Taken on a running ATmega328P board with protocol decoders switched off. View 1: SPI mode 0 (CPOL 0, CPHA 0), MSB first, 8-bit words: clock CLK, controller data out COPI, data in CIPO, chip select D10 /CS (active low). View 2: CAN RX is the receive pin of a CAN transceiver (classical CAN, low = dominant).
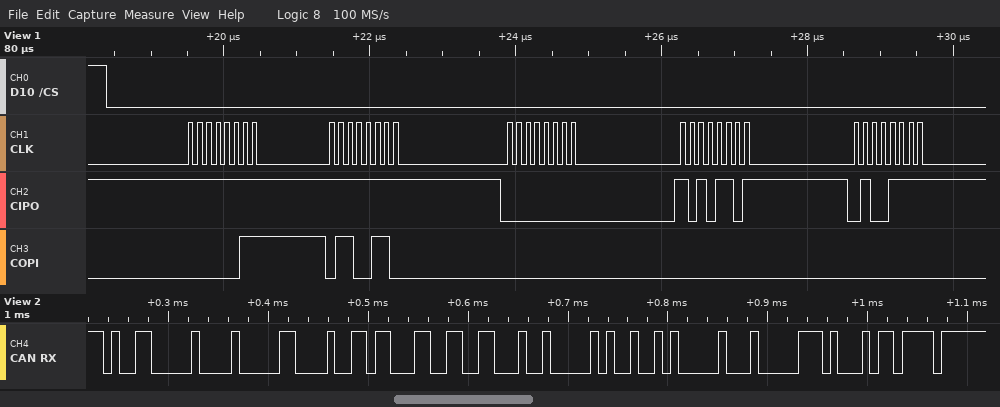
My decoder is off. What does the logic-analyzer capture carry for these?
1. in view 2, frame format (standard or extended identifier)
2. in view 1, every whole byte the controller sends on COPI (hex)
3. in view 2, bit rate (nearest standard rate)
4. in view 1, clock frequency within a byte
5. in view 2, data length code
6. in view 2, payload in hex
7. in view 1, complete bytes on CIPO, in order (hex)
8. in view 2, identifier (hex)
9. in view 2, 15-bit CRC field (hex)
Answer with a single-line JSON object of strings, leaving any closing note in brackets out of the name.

{"in view 2, frame format": "standard", "in view 1, every whole byte the controller sends on COPI": "0x03 0x66 0x00 0x00 0x00", "in view 2, bit rate": "125 kbit/s", "in view 1, clock frequency within a byte": "8 MHz", "in view 2, data length code": "8", "in view 2, payload in hex": "21 36 33 31 20 49 40 20", "in view 1, complete bytes on CIPO, in order": "0xFF 0xFF 0x00 0xAD 0x4F", "in view 2, identifier": "0x4C0", "in view 2, 15-bit CRC field": "0x68B7"}
